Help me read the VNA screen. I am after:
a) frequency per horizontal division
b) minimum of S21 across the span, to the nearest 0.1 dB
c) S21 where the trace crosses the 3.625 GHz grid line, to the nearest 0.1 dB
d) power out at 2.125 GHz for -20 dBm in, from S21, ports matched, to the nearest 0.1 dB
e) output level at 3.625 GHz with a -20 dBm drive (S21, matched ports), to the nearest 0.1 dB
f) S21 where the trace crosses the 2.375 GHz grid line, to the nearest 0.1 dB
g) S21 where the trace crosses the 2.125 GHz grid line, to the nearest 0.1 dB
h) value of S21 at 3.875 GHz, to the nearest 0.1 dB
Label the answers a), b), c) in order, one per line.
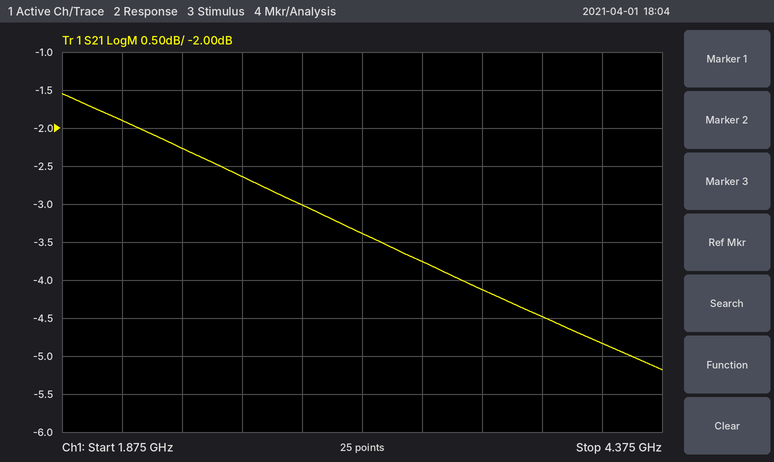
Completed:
a) 250 MHz
b) -5.2 dB
c) -4.1 dB
d) -21.9 dBm
e) -24.1 dBm
f) -2.3 dB
g) -1.9 dB
h) -4.5 dB
